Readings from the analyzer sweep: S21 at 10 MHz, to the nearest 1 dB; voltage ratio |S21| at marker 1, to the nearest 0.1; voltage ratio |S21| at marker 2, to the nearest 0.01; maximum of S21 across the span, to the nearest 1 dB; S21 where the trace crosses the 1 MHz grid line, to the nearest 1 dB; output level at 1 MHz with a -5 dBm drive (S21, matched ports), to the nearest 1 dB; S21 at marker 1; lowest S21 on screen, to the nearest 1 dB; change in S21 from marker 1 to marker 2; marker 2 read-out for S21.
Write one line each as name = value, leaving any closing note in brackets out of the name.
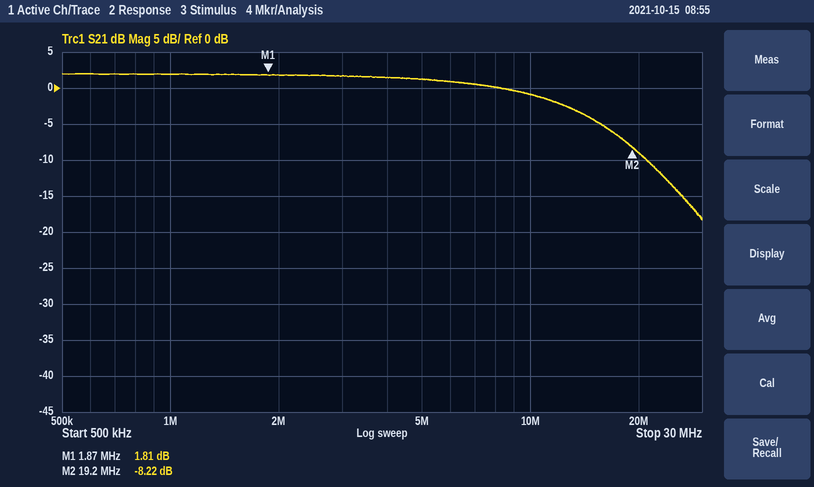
S21 at 10 MHz, to the nearest 1 dB = -1 dB
voltage ratio |S21| at marker 1, to the nearest 0.1 = 1.2
voltage ratio |S21| at marker 2, to the nearest 0.01 = 0.39
maximum of S21 across the span, to the nearest 1 dB = 2 dB
S21 where the trace crosses the 1 MHz grid line, to the nearest 1 dB = 2 dB
output level at 1 MHz with a -5 dBm drive (S21, matched ports), to the nearest 1 dB = -3 dBm
S21 at marker 1 = 1.81 dB
lowest S21 on screen, to the nearest 1 dB = -18 dB
change in S21 from marker 1 to marker 2 = -10.03 dB
marker 2 read-out for S21 = -8.22 dB
